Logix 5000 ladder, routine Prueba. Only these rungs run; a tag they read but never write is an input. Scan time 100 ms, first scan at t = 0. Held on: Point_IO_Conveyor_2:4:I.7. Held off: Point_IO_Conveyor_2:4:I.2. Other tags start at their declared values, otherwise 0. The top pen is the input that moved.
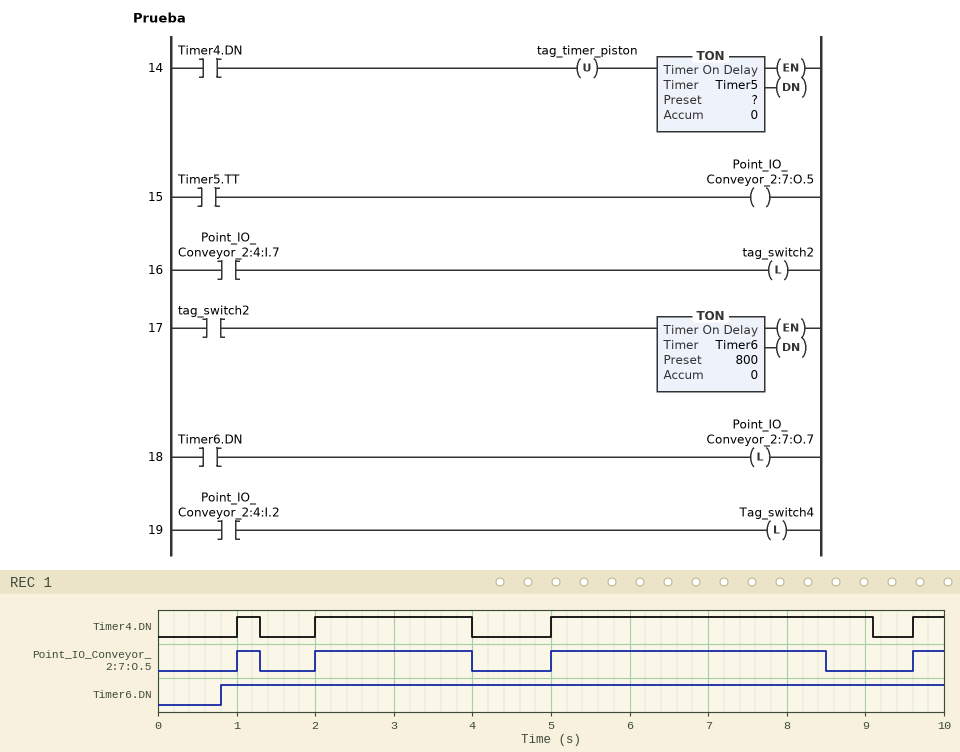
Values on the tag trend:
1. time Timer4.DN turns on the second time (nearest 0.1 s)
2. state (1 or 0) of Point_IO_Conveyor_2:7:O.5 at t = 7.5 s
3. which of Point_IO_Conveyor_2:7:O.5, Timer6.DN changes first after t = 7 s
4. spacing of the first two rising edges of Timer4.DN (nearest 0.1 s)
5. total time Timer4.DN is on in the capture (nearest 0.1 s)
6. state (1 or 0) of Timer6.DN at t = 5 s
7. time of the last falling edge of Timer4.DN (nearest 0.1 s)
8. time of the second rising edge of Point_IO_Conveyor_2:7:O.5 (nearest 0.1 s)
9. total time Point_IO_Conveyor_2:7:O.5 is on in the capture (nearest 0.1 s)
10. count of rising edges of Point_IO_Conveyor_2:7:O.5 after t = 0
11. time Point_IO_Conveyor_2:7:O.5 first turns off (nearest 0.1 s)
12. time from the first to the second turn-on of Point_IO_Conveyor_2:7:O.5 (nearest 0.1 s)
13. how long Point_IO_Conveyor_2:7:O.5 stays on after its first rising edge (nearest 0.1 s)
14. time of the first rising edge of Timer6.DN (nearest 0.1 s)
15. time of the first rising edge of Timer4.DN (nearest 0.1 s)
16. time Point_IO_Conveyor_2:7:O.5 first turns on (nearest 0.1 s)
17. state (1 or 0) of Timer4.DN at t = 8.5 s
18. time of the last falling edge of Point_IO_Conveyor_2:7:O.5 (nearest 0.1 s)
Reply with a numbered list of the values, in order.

1. 2.0 s
2. 1
3. Point_IO_Conveyor_2:7:O.5
4. 1.0 s
5. 6.8 s
6. 1
7. 9.1 s
8. 2.0 s
9. 6.2 s
10. 4
11. 1.3 s
12. 1.0 s
13. 0.3 s
14. 0.8 s
15. 1.0 s
16. 1.0 s
17. 1
18. 8.5 s
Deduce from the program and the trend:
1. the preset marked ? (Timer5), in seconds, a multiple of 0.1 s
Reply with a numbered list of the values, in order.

1. 3.5 s
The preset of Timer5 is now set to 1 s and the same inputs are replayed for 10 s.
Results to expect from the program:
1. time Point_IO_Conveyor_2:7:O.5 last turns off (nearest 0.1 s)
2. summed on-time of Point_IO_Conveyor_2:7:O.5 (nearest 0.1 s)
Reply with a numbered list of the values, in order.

1. 6.0 s
2. 2.7 s
